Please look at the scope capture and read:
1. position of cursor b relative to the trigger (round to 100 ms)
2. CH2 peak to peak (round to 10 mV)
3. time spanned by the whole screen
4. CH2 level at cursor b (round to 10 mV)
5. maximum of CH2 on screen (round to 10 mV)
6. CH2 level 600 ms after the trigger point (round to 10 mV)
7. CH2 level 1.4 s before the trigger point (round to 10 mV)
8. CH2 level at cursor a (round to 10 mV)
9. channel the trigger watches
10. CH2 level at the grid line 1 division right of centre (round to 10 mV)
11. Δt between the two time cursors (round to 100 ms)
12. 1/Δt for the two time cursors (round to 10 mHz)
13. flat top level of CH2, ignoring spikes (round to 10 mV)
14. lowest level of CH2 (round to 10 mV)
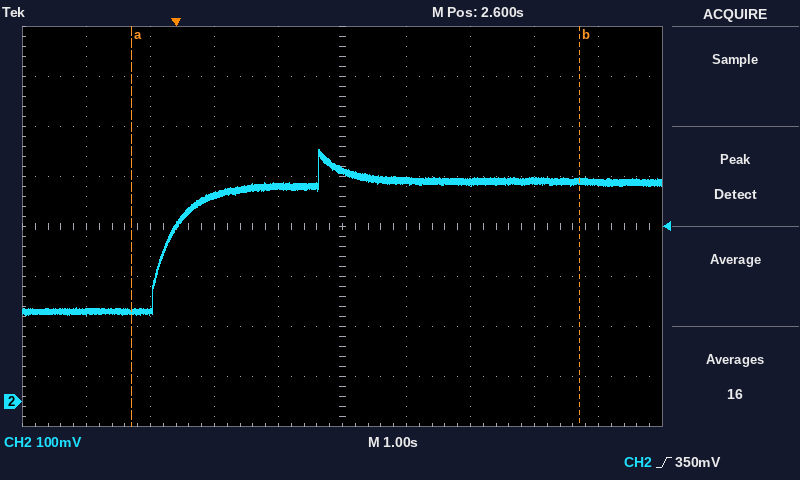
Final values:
+6.3 s
330 mV
10 s
440 mV
500 mV
410 mV
180 mV
180 mV
CH2
440 mV
7.0 s
140 mHz
440 mV
170 mV
